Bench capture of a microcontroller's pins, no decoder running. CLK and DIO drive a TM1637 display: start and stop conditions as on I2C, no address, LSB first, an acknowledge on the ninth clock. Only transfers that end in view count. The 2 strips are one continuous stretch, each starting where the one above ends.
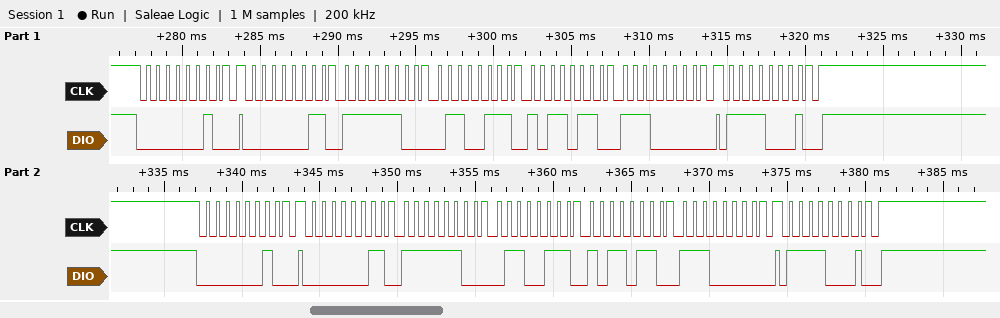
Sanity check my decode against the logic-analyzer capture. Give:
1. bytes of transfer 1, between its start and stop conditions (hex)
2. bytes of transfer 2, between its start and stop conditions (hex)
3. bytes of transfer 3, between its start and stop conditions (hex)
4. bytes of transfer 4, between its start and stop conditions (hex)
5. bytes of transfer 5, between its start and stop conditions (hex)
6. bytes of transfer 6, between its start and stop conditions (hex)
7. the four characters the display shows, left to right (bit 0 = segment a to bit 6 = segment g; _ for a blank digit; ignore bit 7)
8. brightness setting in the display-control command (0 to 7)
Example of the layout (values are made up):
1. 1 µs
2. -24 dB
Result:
1. 40
2. C0 3F E6 6D 07
3. 8F
4. 40
5. C0 3F E6 6D 07
6. 8F
7. 0457
8. 7
